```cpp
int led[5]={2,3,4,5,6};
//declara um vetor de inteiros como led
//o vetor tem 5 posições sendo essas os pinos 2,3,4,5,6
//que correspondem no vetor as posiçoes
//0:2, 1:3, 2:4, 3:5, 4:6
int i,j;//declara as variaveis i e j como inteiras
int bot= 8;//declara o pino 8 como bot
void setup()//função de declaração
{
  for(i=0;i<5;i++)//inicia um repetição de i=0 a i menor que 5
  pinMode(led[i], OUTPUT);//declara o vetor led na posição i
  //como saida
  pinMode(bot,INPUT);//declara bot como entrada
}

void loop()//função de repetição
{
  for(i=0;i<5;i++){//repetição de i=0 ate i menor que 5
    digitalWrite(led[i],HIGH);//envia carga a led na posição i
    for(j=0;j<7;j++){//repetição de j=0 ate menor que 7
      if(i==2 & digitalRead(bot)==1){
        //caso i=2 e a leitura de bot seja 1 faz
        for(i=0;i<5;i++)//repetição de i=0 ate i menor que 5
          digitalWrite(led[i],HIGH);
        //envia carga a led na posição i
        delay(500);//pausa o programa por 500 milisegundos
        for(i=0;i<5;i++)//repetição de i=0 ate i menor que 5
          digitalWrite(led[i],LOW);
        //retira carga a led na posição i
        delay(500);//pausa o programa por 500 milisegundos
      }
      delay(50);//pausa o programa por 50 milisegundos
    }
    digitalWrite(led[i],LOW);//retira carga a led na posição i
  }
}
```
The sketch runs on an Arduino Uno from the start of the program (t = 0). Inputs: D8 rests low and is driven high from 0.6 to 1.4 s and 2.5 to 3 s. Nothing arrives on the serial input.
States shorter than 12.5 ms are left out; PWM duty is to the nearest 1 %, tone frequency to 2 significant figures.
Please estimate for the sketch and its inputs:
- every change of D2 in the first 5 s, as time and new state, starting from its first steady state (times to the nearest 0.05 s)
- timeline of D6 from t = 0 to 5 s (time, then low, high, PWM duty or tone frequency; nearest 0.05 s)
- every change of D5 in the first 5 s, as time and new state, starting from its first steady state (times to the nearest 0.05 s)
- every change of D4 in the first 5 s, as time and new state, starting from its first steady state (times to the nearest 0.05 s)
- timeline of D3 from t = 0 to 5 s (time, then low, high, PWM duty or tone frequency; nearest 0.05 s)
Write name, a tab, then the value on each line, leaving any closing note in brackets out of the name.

every change of D2 in the first 5 s, as time and new state, starting from its first steady state	0 s high; 0.35 s low; 0.7 s high; 1.2 s low; 2.05 s high; 2.4 s low; 2.75 s high; 3.25 s low; 4.1 s high; 4.45 s low
timeline of D6 from t = 0 to 5 s	0 s low; 0.7 s high; 1.2 s low; 2.75 s high; 3.25 s low
every change of D5 in the first 5 s, as time and new state, starting from its first steady state	0 s low; 0.7 s high; 1.2 s low; 2.75 s high; 3.25 s low
every change of D4 in the first 5 s, as time and new state, starting from its first steady state	0 s low; 0.7 s high; 1.2 s low; 2.75 s high; 3.25 s low; 4.8 s high
timeline of D3 from t = 0 to 5 s	0 s low; 0.35 s high; 1.2 s low; 2.4 s high; 3.25 s low; 4.45 s high; 4.8 s low
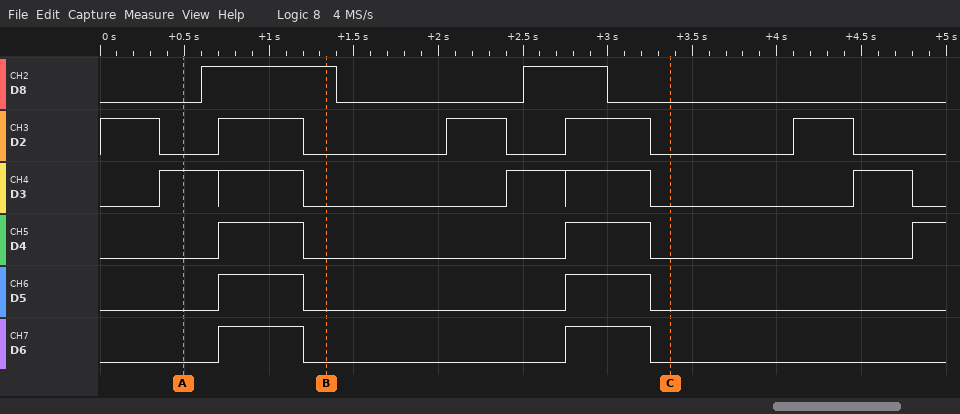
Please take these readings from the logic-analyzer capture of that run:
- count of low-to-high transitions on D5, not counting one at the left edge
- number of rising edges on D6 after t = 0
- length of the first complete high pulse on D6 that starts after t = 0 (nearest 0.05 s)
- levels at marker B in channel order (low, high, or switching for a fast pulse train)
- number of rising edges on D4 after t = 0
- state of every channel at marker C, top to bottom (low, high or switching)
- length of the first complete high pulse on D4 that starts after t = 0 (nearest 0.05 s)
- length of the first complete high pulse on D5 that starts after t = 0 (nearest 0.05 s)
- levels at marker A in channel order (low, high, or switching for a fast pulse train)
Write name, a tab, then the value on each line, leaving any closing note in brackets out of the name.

count of low-to-high transitions on D5, not counting one at the left edge	2
number of rising edges on D6 after t = 0	2
length of the first complete high pulse on D6 that starts after t = 0	0.50 s
levels at marker B in channel order	D8 high, D2 low, D3 low, D4 low, D5 low, D6 low
number of rising edges on D4 after t = 0	3
state of every channel at marker C, top to bottom	D8 low, D2 low, D3 low, D4 low, D5 low, D6 low
length of the first complete high pulse on D4 that starts after t = 0	0.50 s
length of the first complete high pulse on D5 that starts after t = 0	0.50 s
levels at marker A in channel order	D8 low, D2 low, D3 high, D4 low, D5 low, D6 low
